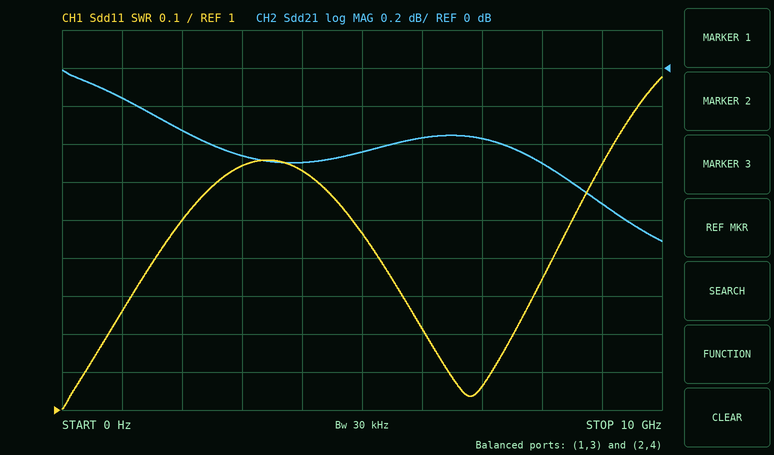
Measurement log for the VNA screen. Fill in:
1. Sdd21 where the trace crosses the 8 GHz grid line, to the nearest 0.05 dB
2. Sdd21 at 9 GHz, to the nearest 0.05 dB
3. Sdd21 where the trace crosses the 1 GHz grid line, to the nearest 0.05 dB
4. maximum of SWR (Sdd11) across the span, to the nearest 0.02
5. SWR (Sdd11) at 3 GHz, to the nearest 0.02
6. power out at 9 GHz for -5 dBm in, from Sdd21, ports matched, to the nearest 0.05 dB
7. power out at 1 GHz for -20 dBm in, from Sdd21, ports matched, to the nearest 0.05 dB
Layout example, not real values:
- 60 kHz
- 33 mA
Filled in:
- -0.50 dB
- -0.70 dB
- -0.15 dB
- 1.88
- 1.64
- -5.70 dBm
- -20.15 dBm
